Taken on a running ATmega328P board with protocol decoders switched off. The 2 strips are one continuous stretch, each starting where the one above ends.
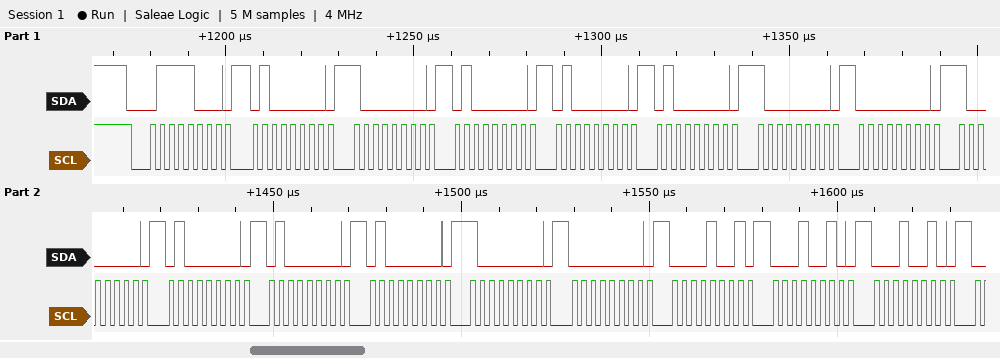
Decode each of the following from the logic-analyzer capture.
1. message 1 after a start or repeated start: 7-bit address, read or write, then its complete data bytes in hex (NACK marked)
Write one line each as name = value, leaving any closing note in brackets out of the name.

message 1 after a start or repeated start: 7-bit address, read or write, then its complete data bytes in hex = 0x3C write: 40 80 40 40 40 80 00 80 40 40 40 80 00 09 12 12
